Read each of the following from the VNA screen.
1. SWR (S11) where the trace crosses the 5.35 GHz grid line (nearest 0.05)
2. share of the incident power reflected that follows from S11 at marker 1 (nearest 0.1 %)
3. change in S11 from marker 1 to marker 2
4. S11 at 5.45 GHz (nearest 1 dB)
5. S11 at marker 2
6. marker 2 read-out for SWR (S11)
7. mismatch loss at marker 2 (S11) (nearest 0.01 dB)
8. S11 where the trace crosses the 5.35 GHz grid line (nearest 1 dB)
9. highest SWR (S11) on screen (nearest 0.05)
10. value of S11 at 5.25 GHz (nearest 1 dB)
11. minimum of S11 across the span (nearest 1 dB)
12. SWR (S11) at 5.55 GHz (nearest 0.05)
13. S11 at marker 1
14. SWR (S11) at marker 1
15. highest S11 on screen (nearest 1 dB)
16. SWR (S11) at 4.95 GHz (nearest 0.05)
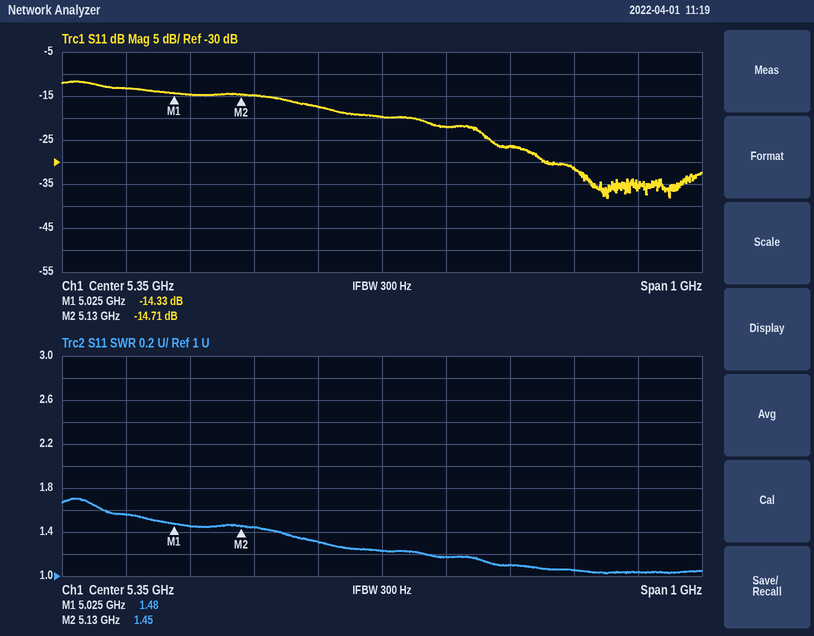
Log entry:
1.25
3.7 %
-0.38 dB
-22 dB
-14.71 dB
1.45
0.15 dB
-20 dB
1.70
-17 dB
-38 dB
1.10
-14.33 dB
1.48
-12 dB
1.55
